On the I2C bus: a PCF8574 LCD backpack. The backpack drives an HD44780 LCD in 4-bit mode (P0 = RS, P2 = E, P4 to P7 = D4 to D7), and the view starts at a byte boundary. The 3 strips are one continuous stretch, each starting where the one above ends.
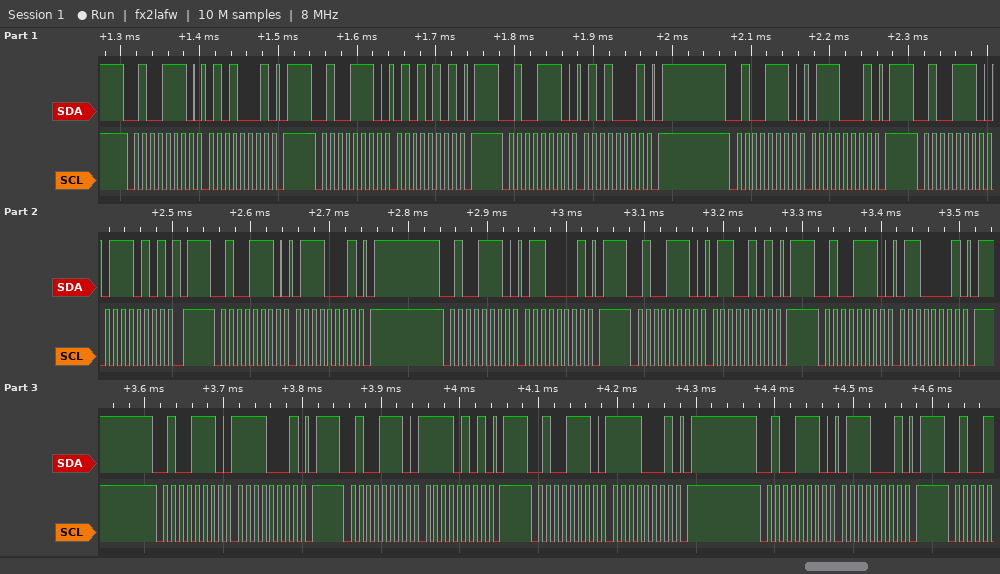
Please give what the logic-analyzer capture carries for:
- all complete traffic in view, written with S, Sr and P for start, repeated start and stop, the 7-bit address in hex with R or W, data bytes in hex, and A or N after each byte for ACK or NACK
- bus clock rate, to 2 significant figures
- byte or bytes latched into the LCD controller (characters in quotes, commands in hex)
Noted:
S 27W A 51 A P S 27W A 55 A P S 27W A 51 A P S 27W A 71 A P S 27W A 75 A P S 27W A 71 A P S 27W A 61 A P S 27W A 65 A P S 27W A 61 A P S 27W A F1 A P S 27W A F5 A P S 27W A F1 A P S 27W A 71 A P
100 kHz
'W' 'o'
